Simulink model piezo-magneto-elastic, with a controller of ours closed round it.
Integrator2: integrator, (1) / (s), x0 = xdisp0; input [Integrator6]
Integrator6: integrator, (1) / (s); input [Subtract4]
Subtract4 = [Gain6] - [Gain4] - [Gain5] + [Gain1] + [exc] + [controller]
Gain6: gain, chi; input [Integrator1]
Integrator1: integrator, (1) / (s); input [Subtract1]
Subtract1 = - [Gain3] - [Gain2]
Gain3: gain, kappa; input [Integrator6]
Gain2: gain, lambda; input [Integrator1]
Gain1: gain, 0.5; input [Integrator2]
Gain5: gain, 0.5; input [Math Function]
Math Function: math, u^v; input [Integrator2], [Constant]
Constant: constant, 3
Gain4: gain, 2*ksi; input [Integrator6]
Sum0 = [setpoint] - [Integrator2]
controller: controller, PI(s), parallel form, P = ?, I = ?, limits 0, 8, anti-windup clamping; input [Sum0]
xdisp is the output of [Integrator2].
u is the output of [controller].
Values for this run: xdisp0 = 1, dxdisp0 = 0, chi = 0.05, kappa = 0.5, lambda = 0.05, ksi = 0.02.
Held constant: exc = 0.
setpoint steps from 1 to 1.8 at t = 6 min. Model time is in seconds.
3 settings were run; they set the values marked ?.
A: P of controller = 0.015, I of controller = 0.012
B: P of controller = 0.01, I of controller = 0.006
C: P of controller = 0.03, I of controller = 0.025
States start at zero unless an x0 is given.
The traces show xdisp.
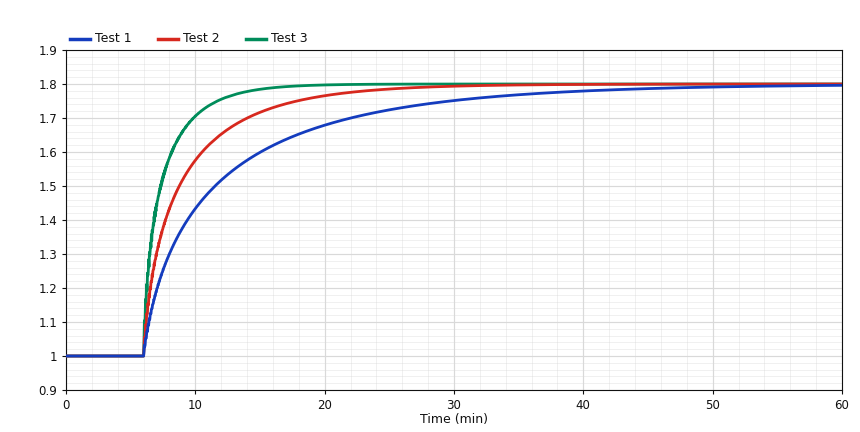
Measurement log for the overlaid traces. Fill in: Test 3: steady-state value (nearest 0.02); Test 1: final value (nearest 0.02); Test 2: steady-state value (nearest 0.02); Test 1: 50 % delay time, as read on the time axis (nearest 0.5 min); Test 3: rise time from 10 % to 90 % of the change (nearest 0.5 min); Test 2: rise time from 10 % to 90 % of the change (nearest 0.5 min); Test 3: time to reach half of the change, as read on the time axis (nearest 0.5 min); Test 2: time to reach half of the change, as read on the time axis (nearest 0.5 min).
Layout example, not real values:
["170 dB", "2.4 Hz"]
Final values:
["1.80", "1.80", "1.80", "9.5 min", "4.5 min", "9.0 min", "7.0 min", "7.5 min"]
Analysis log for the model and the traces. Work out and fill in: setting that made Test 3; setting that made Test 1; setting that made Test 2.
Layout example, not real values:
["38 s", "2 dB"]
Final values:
["C", "B", "A"]
